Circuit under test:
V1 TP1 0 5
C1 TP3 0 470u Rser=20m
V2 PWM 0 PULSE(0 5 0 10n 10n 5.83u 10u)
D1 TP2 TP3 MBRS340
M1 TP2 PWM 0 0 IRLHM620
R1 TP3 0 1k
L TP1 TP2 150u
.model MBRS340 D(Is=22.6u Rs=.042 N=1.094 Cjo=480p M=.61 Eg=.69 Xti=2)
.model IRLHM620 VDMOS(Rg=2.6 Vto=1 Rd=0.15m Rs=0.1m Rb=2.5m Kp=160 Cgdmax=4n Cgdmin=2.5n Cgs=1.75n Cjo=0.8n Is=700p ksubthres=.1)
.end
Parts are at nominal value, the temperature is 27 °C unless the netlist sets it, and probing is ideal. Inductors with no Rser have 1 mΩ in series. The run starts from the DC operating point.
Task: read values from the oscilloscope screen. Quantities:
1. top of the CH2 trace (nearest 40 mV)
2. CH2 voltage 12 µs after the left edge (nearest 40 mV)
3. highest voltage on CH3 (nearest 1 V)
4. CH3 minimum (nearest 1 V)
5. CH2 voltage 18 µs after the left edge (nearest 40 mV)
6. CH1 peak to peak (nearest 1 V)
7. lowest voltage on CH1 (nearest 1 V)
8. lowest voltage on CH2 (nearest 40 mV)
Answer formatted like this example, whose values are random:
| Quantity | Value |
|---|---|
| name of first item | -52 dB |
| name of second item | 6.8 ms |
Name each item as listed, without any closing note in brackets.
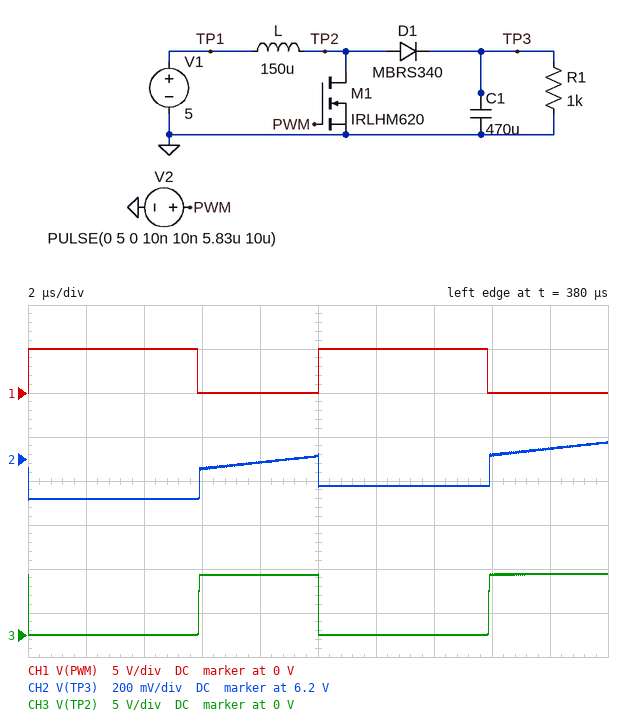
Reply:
| Quantity | Value |
|---|---|
| top of the CH2 trace | 6.28 V |
| CH2 voltage 12 µs after the left edge | 6.08 V |
| highest voltage on CH3 | 7 V |
| CH3 minimum | 0 V |
| CH2 voltage 18 µs after the left edge | 6.24 V |
| CH1 peak to peak | 5 V |
| lowest voltage on CH1 | 0 V |
| lowest voltage on CH2 | 6.00 V |
